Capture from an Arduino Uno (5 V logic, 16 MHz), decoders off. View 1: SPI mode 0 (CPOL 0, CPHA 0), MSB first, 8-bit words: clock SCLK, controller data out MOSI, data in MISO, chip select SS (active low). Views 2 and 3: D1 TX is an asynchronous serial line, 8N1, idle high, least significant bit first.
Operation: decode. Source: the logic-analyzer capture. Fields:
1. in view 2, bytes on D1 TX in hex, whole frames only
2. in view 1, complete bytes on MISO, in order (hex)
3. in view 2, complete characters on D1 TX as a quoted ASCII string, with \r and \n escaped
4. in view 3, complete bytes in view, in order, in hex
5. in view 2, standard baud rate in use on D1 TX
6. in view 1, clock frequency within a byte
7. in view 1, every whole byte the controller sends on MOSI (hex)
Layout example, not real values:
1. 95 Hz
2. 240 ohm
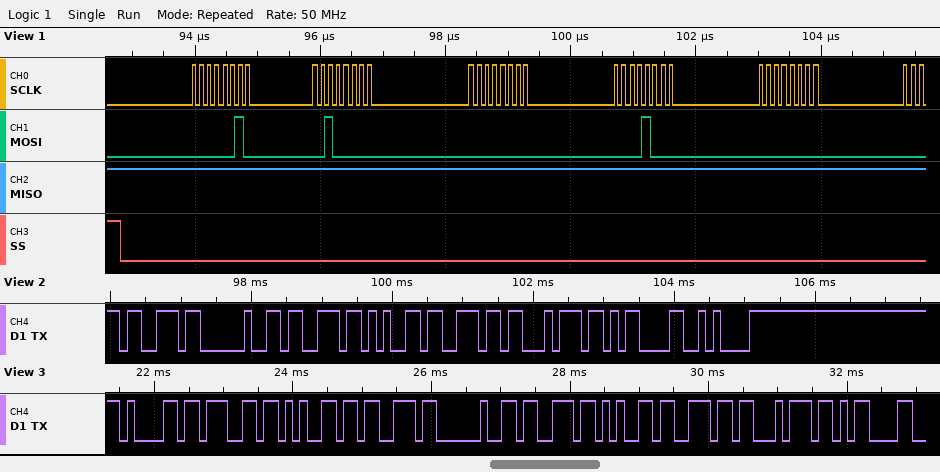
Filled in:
1. 73 20 73 65 6E 74 0D 0A
2. FF FF FF FF FF
3. "s sent\r\n"
4. 0x61 0x67 0x65 0x73 0x20 0x73 0x65 0x6E 0x74 0x0D
5. 9600 baud
6. 8 MHz
7. 02 20 00 08 00
